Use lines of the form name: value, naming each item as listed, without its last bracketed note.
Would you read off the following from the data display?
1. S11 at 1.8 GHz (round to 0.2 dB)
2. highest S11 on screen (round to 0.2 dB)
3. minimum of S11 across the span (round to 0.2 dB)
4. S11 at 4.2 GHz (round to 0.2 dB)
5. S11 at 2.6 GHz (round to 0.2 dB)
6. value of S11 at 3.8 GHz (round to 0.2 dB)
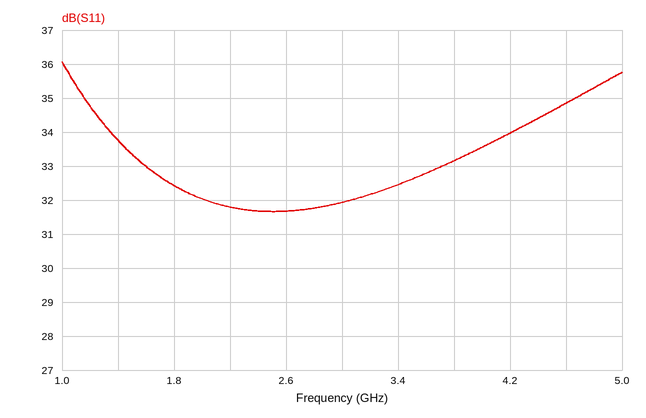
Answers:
S11 at 1.8 GHz: 32.4 dB
highest S11 on screen: 36.0 dB
minimum of S11 across the span: 31.6 dB
S11 at 4.2 GHz: 34.0 dB
S11 at 2.6 GHz: 31.6 dB
value of S11 at 3.8 GHz: 33.2 dB
